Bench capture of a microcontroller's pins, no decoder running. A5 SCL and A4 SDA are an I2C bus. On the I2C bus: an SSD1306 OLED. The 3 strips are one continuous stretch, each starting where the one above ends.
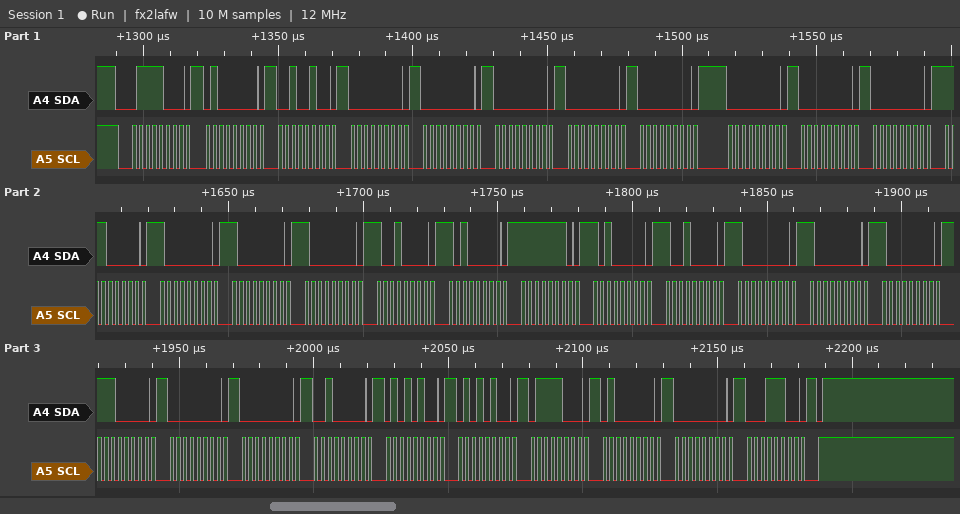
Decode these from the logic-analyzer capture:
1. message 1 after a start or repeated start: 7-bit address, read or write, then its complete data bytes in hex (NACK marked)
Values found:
0x3C write: 40 24 00 00 00 00 00 00 00 00 E0 80 80 80 90 A0 FE A0 90 80 80 80 E0 00 00 20 54 54 78 40 00 1C
